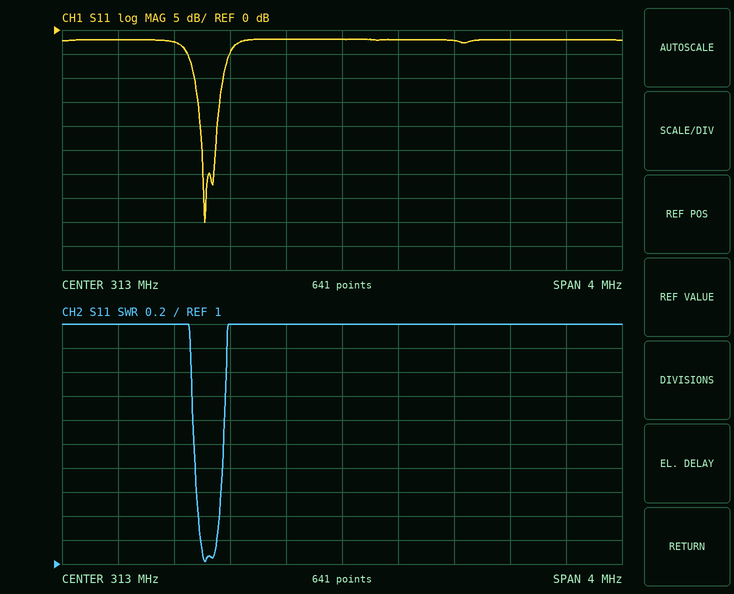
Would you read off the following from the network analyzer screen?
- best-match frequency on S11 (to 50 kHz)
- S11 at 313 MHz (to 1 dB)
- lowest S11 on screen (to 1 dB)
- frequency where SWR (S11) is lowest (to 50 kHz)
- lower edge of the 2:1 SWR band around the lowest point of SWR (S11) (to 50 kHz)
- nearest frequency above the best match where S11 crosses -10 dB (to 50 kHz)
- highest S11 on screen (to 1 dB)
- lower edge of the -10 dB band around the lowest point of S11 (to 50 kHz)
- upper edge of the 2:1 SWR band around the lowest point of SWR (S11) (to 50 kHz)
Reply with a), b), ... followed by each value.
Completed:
a) 312.00 MHz
b) -2 dB
c) -40 dB
d) 312.00 MHz
e) 311.95 MHz
f) 312.15 MHz
g) -2 dB
h) 311.95 MHz
i) 312.15 MHz
